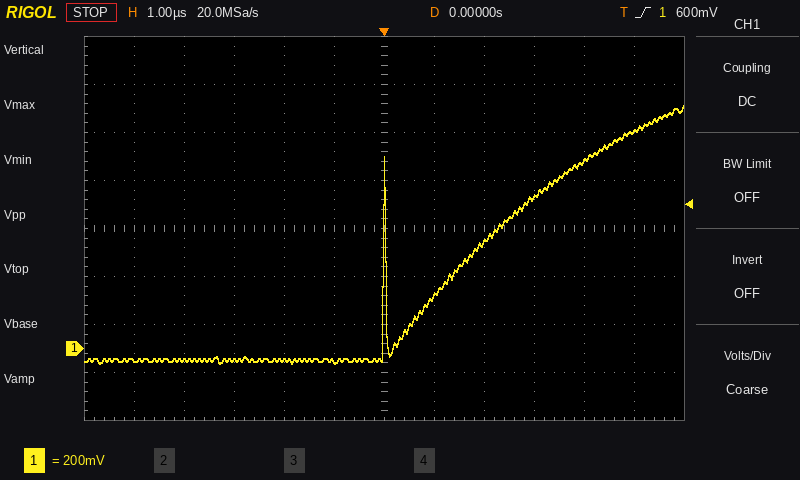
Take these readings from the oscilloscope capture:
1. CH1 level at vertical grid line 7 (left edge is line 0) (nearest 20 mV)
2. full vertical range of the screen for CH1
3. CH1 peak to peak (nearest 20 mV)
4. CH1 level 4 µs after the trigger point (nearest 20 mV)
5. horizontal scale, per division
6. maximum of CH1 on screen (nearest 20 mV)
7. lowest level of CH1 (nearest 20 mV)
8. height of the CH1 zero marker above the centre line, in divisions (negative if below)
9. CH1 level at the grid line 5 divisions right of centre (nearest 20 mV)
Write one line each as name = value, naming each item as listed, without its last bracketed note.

CH1 level at vertical grid line 7 (left edge is line 0) = 220 mV
full vertical range of the screen for CH1 = 1.6 V
CH1 peak to peak = 1.08 V
CH1 level 4 µs after the trigger point = 780 mV
horizontal scale, per division = 1 µs
maximum of CH1 on screen = 1.02 V
lowest level of CH1 = -60 mV
height of the CH1 zero marker above the centre line, in divisions = -2.5 div
CH1 level at the grid line 5 divisions right of centre = 900 mV
